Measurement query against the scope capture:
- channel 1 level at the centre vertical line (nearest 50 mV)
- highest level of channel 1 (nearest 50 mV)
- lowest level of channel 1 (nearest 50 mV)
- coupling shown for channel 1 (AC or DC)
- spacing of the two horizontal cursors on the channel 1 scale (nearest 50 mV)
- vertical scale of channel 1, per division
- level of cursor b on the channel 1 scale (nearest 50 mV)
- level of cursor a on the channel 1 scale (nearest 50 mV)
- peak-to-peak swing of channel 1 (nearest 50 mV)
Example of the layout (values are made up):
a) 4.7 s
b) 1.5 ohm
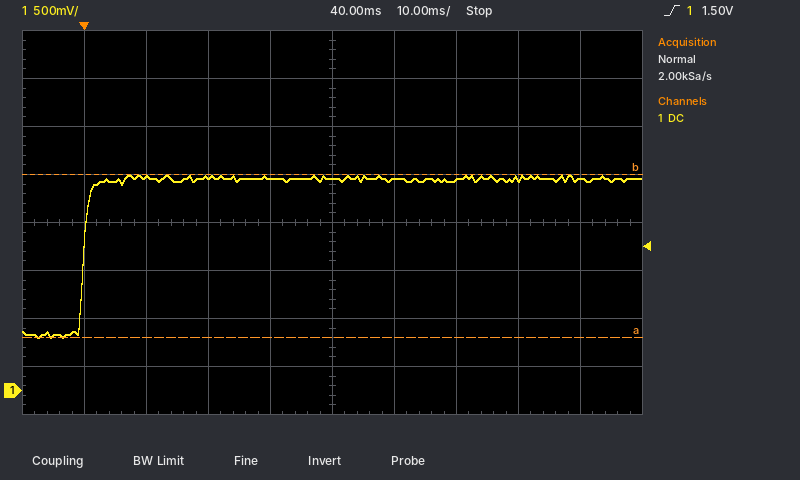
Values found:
a) 2.20 V
b) 2.25 V
c) 550 mV
d) DC
e) 1.70 V
f) 500 mV
g) 2.25 V
h) 550 mV
i) 1.70 V
